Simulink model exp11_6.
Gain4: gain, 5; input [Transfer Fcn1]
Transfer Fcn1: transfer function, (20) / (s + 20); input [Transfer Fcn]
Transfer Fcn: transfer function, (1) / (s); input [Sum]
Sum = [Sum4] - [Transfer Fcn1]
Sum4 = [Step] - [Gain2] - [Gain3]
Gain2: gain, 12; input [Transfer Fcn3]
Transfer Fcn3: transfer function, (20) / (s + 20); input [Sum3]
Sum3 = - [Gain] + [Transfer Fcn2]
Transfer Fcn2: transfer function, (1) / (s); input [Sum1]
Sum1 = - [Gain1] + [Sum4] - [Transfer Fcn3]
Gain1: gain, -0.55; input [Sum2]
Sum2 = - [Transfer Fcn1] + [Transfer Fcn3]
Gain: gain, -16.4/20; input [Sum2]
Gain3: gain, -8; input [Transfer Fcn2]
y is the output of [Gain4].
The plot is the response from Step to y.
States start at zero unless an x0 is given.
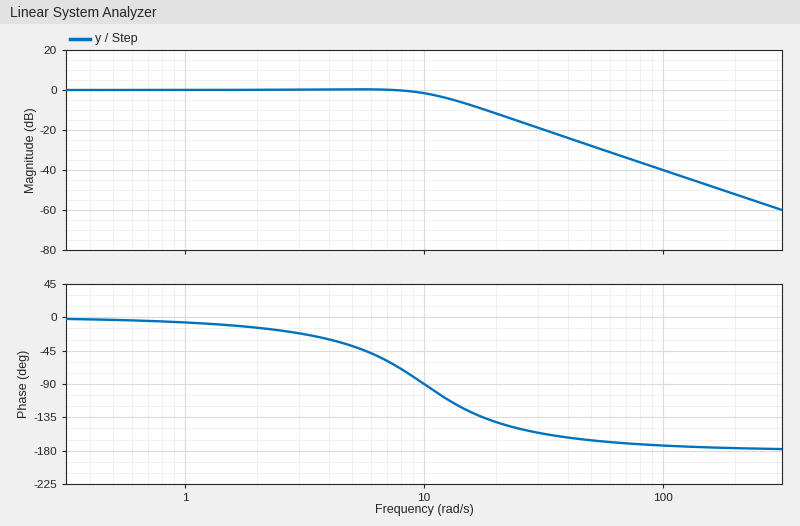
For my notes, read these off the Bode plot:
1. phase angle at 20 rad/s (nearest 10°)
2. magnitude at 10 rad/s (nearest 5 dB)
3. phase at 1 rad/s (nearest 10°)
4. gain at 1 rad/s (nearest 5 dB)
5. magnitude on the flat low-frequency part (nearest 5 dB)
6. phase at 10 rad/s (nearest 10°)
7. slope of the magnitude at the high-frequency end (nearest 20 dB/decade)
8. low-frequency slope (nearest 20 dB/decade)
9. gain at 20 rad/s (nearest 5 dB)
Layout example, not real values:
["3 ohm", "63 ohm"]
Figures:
["-140°", "0 dB", "-10°", "0 dB", "0 dB", "-90°", "-40 dB/decade", "0 dB/decade", "-10 dB"]
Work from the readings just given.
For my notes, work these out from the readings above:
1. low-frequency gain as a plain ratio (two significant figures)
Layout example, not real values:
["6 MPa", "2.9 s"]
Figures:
["1.0"]
